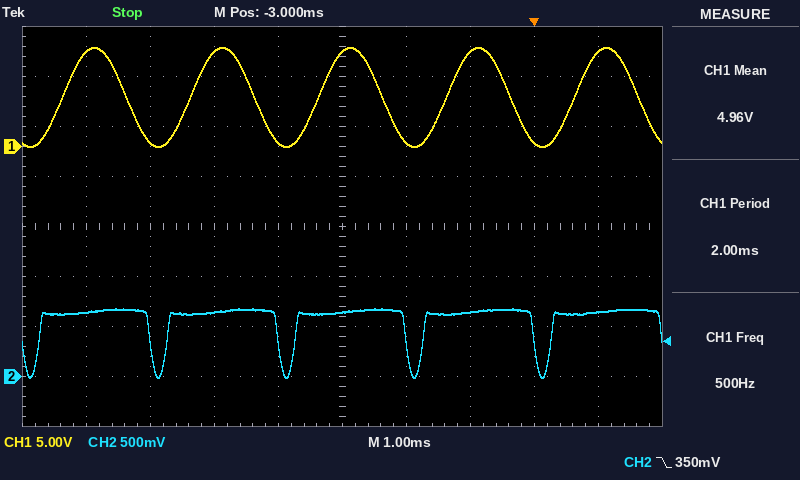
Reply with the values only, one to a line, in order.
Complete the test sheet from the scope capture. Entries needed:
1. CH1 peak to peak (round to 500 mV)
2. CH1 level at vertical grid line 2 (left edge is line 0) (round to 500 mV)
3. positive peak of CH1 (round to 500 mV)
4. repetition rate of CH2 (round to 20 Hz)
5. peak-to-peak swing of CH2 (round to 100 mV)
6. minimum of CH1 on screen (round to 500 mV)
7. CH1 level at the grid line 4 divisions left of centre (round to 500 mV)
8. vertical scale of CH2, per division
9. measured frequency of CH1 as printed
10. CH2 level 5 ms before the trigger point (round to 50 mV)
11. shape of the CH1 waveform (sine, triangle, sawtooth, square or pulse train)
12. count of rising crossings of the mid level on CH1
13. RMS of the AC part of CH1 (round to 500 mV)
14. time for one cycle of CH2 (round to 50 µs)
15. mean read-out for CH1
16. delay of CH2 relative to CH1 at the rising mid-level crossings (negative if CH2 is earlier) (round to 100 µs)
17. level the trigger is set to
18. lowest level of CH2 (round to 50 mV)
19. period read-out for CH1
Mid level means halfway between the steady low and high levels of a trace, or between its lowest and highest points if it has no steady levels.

10.0 V
500 mV
10.0 V
500 Hz
700 mV
0.0 V
9.5 V
500 mV
500 Hz
650 mV
sine
5
3.5 V
2.00 ms
4.96 V
-400 µs
350 mV
0 mV
2.00 ms
